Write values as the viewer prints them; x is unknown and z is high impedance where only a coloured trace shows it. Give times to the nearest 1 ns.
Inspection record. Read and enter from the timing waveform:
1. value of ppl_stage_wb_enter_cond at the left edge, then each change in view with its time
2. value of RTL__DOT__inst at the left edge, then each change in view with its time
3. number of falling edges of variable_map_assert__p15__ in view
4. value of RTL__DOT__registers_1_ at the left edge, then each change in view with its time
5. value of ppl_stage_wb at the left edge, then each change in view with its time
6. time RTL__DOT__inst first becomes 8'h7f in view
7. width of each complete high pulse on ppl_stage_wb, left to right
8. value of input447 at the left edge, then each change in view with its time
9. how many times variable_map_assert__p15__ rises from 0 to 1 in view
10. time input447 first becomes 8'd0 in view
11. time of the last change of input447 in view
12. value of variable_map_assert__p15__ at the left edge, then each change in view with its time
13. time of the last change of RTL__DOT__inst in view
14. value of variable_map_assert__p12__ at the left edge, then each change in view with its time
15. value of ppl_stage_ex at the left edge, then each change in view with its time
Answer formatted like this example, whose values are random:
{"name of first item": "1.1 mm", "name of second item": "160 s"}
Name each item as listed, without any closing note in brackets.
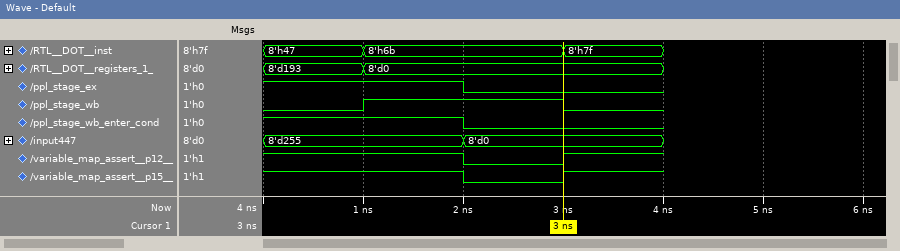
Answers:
{"value of ppl_stage_wb_enter_cond at the left edge, then each change in view with its time": "1, 0 at 2 ns", "value of RTL__DOT__inst at the left edge, then each change in view with its time": "8'h47, 8'h6b at 1 ns, 8'h7f at 3 ns", "number of falling edges of variable_map_assert__p15__ in view": "1", "value of RTL__DOT__registers_1_ at the left edge, then each change in view with its time": "8'd193, 8'd0 at 1 ns", "value of ppl_stage_wb at the left edge, then each change in view with its time": "0, 1 at 1 ns, 0 at 3 ns", "time RTL__DOT__inst first becomes 8'h7f in view": "3 ns", "width of each complete high pulse on ppl_stage_wb, left to right": "2 ns", "value of input447 at the left edge, then each change in view with its time": "8'd255, 8'd0 at 2 ns", "how many times variable_map_assert__p15__ rises from 0 to 1 in view": "1", "time input447 first becomes 8'd0 in view": "2 ns", "time of the last change of input447 in view": "2 ns", "value of variable_map_assert__p15__ at the left edge, then each change in view with its time": "1, 0 at 2 ns, 1 at 3 ns", "time of the last change of RTL__DOT__inst in view": "3 ns", "value of variable_map_assert__p12__ at the left edge, then each change in view with its time": "1, 0 at 2 ns, 1 at 3 ns", "value of ppl_stage_ex at the left edge, then each change in view with its time": "1, 0 at 2 ns"}
